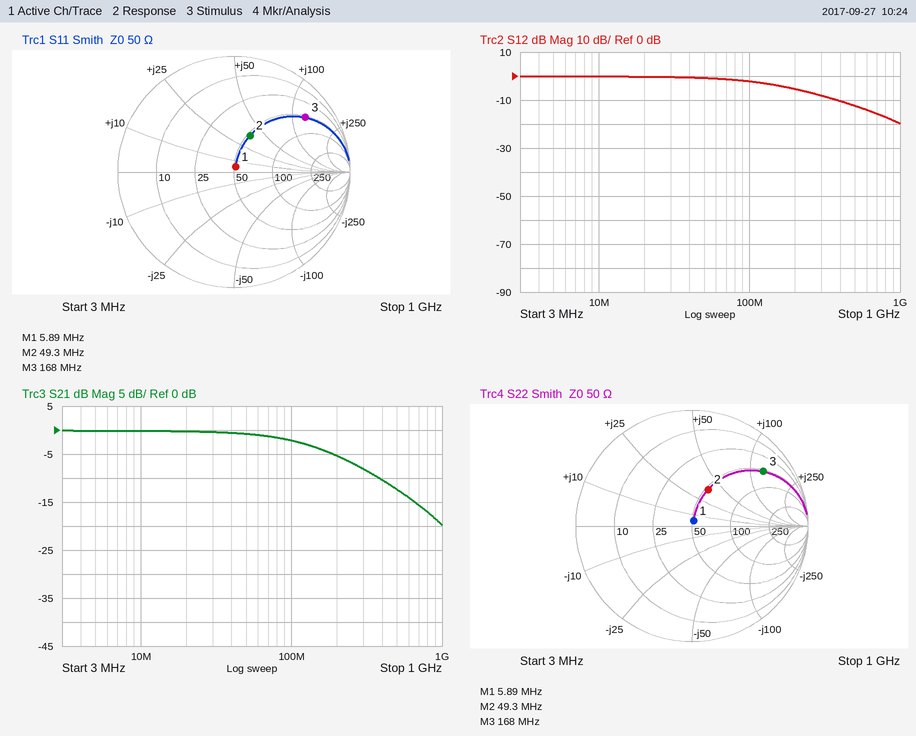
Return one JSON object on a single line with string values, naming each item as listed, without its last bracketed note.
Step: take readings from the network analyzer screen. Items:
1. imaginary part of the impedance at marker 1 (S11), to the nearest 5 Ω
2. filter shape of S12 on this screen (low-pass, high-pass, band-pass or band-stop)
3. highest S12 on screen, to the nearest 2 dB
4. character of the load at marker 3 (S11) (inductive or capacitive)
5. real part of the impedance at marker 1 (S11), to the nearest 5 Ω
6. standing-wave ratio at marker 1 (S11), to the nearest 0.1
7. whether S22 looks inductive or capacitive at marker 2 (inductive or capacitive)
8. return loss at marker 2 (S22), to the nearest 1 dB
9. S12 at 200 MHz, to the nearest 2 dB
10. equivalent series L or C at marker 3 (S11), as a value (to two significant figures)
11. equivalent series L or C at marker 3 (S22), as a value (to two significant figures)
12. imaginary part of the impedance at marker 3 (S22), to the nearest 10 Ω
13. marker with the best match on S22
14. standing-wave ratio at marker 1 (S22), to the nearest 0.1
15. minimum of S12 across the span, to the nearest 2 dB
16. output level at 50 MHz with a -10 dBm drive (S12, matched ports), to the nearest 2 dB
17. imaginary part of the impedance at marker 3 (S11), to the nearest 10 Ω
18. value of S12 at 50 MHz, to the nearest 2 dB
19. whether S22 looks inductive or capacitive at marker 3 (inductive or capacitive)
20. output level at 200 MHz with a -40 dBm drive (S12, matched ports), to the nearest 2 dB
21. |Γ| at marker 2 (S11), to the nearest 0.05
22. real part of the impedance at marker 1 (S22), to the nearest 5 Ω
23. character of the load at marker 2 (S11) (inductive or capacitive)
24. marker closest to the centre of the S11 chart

{"imaginary part of the impedance at marker 1 (S11), to the nearest 5 Ω": "+5 Ω", "filter shape of S12 on this screen": "low-pass", "highest S12 on screen, to the nearest 2 dB": "0 dB", "character of the load at marker 3 (S11)": "inductive", "real part of the impedance at marker 1 (S11), to the nearest 5 Ω": "50 Ω", "standing-wave ratio at marker 1 (S11), to the nearest 0.1": "1.1", "whether S22 looks inductive or capacitive at marker 2": "inductive", "return loss at marker 2 (S22), to the nearest 1 dB": "9 dB", "S12 at 200 MHz, to the nearest 2 dB": "-6 dB", "equivalent series L or C at marker 3 (S11), as a value": "120 nH", "equivalent series L or C at marker 3 (S22), as a value": "120 nH", "imaginary part of the impedance at marker 3 (S22), to the nearest 10 Ω": "+130 Ω", "marker with the best match on S22": "marker 1", "standing-wave ratio at marker 1 (S22), to the nearest 0.1": "1.1", "minimum of S12 across the span, to the nearest 2 dB": "-20 dB", "output level at 50 MHz with a -10 dBm drive (S12, matched ports), to the nearest 2 dB": "-10 dBm", "imaginary part of the impedance at marker 3 (S11), to the nearest 10 Ω": "+130 Ω", "value of S12 at 50 MHz, to the nearest 2 dB": "0 dB", "whether S22 looks inductive or capacitive at marker 3": "inductive", "output level at 200 MHz with a -40 dBm drive (S12, matched ports), to the nearest 2 dB": "-46 dBm", "|Γ| at marker 2 (S11), to the nearest 0.05": "0.35", "real part of the impedance at marker 1 (S22), to the nearest 5 Ω": "50 Ω", "character of the load at marker 2 (S11)": "inductive", "marker closest to the centre of the S11 chart": "marker 1"}
